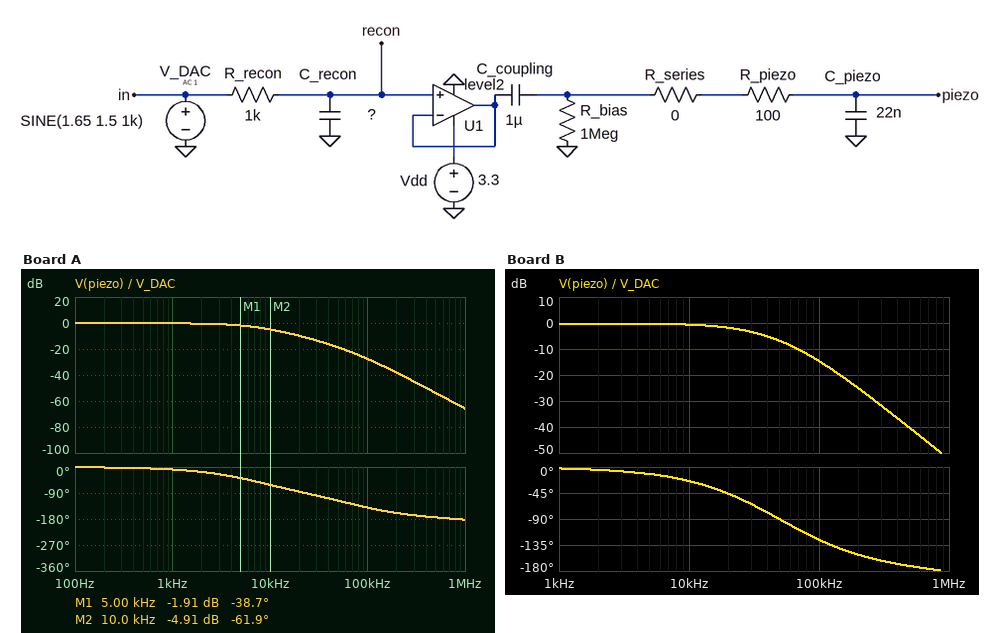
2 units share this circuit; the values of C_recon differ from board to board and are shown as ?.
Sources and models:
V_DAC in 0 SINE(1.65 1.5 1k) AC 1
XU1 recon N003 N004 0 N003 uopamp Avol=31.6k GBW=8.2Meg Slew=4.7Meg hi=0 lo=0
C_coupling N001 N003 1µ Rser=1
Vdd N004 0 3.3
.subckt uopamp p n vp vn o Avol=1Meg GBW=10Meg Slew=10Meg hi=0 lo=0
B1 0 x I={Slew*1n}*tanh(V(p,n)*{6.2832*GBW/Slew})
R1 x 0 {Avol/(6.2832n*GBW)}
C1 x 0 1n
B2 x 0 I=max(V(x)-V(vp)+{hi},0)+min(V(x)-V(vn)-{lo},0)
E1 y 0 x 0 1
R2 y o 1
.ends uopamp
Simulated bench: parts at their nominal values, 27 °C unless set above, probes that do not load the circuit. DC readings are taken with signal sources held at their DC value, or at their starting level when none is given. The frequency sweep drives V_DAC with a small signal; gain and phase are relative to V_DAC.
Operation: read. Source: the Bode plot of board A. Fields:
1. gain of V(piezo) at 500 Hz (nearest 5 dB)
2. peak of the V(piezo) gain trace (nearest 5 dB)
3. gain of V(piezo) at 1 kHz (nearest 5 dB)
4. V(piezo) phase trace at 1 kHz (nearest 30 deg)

0 dB
0 dB
0 dB
0 deg
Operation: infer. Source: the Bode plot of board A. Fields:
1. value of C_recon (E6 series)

22 nF
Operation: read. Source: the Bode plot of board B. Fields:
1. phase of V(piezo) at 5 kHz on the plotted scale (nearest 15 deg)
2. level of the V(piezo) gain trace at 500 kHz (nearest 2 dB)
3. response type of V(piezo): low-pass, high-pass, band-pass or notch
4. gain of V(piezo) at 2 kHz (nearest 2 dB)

-15 deg
-40 dB
low-pass
0 dB
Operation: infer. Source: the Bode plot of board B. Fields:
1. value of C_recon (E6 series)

4.7 nF
